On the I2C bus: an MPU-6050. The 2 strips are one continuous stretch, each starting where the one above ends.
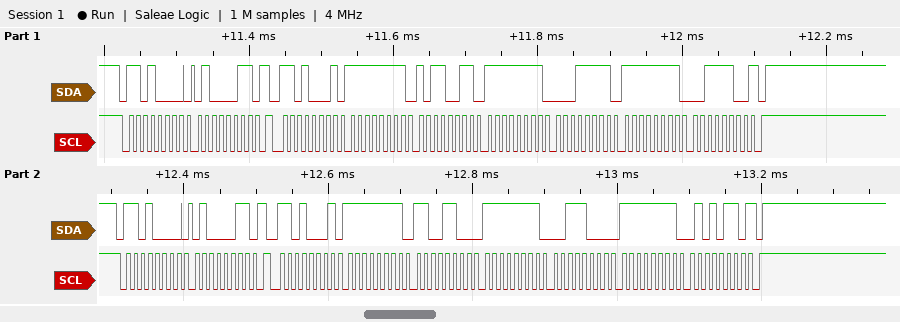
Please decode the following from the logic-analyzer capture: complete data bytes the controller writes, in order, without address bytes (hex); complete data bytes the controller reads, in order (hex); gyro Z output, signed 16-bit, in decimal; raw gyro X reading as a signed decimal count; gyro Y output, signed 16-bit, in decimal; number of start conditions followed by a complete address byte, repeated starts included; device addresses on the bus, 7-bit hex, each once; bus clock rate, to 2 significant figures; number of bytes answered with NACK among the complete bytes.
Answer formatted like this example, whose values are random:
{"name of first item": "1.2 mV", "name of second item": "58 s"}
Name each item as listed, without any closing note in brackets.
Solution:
{"complete data bytes the controller writes, in order, without address bytes": "43 43", "complete data bytes the controller reads, in order": "FF B3 FF 1F FF 3C FF CC FF 38 FF 56", "gyro Z output, signed 16-bit, in decimal": "-196", "raw gyro X reading as a signed decimal count": "-77", "gyro Y output, signed 16-bit, in decimal": "-225", "number of start conditions followed by a complete address byte, repeated starts included": "4", "device addresses on the bus, 7-bit hex, each once": "0x68", "bus clock rate, to 2 significant figures": "100 kHz", "number of bytes answered with NACK among the complete bytes": "2"}
